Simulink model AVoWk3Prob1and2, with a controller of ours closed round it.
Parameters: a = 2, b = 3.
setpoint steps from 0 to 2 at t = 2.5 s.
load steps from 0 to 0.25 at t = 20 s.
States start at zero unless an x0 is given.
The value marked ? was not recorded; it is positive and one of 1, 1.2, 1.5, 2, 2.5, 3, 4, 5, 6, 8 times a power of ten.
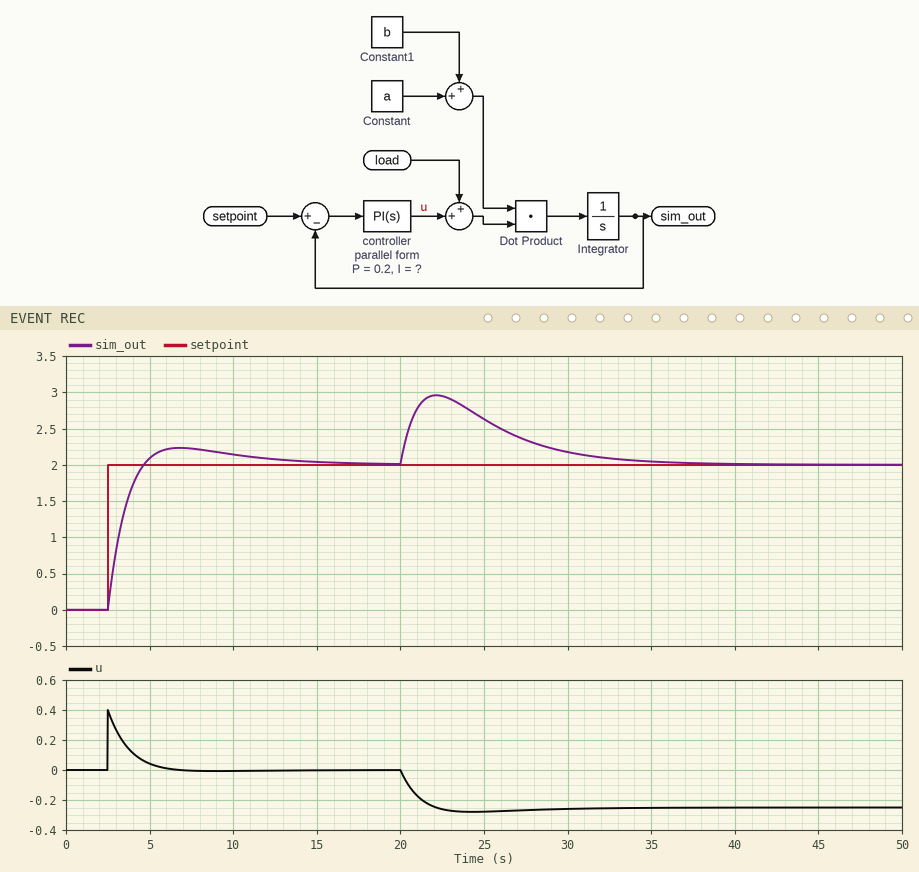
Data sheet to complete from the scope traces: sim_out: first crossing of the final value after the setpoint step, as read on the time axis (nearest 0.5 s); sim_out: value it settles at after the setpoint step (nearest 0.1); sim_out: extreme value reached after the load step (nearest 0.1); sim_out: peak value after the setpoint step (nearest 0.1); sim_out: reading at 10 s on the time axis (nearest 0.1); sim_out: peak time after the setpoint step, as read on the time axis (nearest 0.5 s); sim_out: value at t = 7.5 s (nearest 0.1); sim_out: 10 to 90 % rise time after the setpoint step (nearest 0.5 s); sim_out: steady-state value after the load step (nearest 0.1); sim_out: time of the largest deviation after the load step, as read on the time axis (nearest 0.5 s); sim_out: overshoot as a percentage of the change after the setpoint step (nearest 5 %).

4.5 s
2.0
3.0
2.2
2.1
7.0 s
2.2
1.5 s
2.0
22.0 s
10 %
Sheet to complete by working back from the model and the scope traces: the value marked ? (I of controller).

0.04
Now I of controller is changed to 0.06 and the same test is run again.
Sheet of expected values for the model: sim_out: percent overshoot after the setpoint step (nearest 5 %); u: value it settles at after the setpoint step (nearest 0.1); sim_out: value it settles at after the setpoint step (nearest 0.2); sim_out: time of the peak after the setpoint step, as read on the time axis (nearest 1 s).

15 %
0.0
2.0
6 s
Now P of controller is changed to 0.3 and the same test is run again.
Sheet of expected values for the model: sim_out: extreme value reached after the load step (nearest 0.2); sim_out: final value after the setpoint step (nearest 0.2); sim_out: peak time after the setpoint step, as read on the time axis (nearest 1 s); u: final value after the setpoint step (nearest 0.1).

2.8
2.0
6 s
0.0
